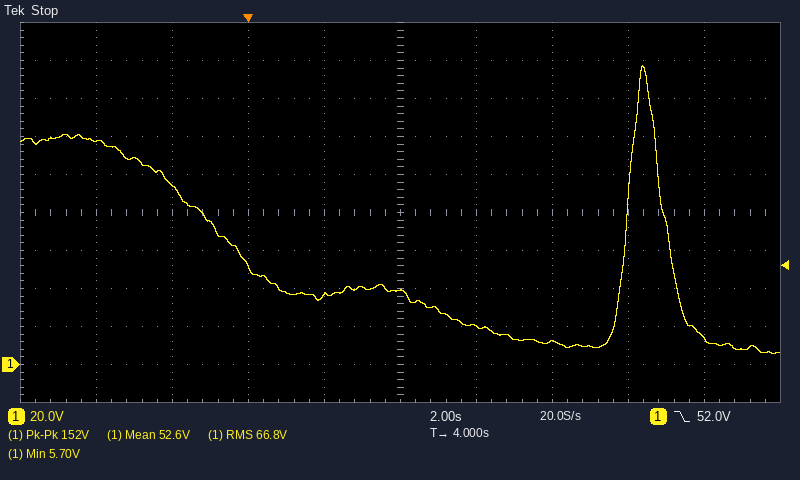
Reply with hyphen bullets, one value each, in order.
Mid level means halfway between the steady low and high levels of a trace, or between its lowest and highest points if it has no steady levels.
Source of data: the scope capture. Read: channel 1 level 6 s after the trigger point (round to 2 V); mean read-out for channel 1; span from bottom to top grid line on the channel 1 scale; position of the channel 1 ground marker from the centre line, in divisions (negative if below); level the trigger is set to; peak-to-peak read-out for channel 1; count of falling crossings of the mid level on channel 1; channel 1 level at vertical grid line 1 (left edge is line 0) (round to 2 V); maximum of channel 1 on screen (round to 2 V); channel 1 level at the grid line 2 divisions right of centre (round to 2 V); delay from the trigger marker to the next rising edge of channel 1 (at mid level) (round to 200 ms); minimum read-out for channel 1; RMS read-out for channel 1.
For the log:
- 20 V
- 52.6 V
- 200 V
- -4.0 div
- 52.0 V
- 152 V
- 2
- 118 V
- 158 V
- 12 V
- 10.0 s
- 5.70 V
- 66.8 V
